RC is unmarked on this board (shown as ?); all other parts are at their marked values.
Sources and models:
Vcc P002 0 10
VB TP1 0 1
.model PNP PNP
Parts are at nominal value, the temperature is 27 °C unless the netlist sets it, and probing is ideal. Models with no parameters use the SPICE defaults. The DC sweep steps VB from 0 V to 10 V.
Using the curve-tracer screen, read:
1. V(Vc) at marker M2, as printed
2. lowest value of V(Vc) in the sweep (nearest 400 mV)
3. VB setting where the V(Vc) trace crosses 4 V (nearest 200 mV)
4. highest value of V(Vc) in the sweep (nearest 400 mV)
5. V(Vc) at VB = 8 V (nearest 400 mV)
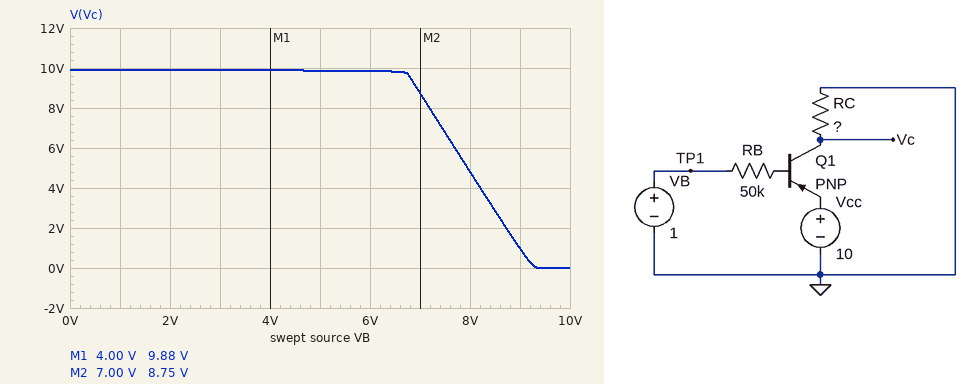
8.75 V
0 V
8.2 V
10.0 V
4.8 V
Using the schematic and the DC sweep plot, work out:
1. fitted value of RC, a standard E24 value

2 kΩ
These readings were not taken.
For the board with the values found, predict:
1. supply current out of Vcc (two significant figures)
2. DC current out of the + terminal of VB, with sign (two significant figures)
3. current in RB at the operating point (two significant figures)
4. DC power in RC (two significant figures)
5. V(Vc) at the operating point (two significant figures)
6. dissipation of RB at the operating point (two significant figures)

5.1 mA
-160 µA
160 µA
49 mW
9.9 V
1.3 mW
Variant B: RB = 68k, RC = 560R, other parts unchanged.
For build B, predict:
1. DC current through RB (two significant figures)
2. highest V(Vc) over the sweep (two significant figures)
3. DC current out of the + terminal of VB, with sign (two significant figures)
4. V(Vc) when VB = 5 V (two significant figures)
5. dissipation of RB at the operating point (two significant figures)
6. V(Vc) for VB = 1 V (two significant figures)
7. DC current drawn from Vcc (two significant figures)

120 µA
7.5 V
-120 µA
3.4 V
980 µW
6.7 V
12 mA
